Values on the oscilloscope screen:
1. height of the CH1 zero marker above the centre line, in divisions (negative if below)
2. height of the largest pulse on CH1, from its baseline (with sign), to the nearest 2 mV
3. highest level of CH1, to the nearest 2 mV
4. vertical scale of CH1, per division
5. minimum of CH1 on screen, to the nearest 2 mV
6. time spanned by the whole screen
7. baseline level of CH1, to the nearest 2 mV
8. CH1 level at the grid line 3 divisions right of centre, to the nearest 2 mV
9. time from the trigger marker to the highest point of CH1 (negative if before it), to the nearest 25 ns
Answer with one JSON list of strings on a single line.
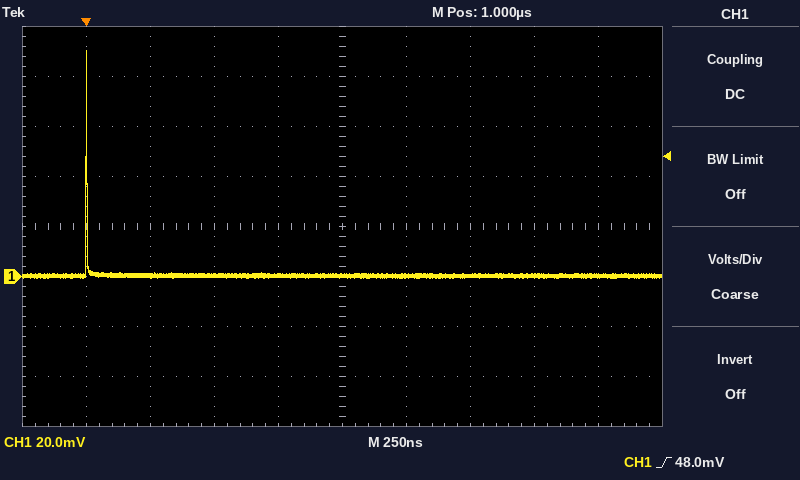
["-1.0 div", "+90 mV", "90 mV", "20 mV", "0 mV", "2.5 µs", "0 mV", "0 mV", "0 ns"]
